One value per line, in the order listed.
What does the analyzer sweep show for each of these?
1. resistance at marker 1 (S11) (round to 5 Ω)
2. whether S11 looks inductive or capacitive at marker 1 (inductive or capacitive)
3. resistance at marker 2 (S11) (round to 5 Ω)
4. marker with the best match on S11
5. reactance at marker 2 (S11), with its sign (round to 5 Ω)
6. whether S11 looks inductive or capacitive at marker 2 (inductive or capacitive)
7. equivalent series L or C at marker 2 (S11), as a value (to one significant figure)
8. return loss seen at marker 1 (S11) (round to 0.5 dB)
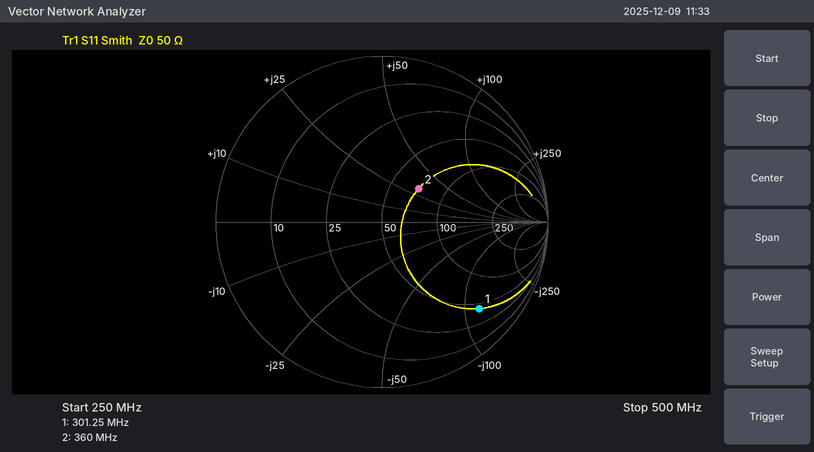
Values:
45 Ω
capacitive
70 Ω
marker 2
+30 Ω
inductive
10 nH
2.0 dB
